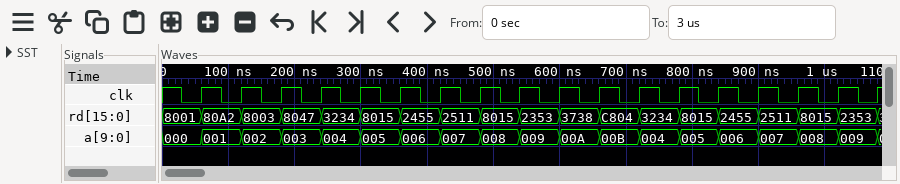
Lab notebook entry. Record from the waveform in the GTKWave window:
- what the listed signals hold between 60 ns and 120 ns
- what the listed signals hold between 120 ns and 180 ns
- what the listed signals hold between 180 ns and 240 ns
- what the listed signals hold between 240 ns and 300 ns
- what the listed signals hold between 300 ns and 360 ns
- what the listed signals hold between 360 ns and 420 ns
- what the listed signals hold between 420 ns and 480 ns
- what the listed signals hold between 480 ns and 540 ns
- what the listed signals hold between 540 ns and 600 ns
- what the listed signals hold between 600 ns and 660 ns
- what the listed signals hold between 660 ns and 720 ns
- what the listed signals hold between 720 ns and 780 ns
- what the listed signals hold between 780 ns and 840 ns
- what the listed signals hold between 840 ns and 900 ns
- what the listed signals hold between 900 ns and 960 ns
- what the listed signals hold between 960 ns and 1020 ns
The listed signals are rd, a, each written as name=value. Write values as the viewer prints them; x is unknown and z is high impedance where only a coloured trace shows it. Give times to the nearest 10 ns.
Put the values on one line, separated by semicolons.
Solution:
rd=80A2, a=001; rd=8003, a=002; rd=8047, a=003; rd=3234, a=004; rd=8015, a=005; rd=2455, a=006; rd=2511, a=007; rd=8015, a=008; rd=2353, a=009; rd=3738, a=00A; rd=C804, a=00B; rd=3234, a=004; rd=8015, a=005; rd=2455, a=006; rd=2511, a=007; rd=8015, a=008
